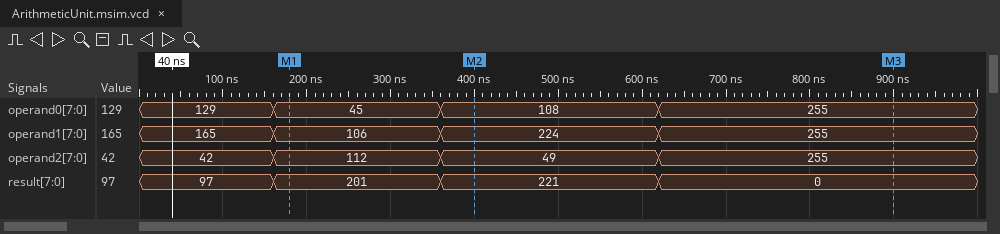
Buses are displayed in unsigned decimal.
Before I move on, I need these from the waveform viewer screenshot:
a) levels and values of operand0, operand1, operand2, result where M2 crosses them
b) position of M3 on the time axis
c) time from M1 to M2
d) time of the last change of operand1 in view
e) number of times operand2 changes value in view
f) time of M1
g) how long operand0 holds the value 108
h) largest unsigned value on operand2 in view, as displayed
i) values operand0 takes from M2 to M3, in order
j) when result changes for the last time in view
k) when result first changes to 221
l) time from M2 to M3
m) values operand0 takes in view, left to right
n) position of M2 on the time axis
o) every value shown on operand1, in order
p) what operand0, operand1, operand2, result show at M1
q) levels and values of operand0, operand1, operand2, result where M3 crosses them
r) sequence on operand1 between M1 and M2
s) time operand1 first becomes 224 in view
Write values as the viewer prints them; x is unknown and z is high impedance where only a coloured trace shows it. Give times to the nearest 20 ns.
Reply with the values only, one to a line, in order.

operand0=108, operand1=224, operand2=49, result=221
900 ns
220 ns
620 ns
3
180 ns
260 ns
255
108, 255
620 ns
360 ns
500 ns
129, 45, 108, 255
400 ns
165, 106, 224, 255
operand0=45, operand1=106, operand2=112, result=201
operand0=255, operand1=255, operand2=255, result=0
106, 224
360 ns
